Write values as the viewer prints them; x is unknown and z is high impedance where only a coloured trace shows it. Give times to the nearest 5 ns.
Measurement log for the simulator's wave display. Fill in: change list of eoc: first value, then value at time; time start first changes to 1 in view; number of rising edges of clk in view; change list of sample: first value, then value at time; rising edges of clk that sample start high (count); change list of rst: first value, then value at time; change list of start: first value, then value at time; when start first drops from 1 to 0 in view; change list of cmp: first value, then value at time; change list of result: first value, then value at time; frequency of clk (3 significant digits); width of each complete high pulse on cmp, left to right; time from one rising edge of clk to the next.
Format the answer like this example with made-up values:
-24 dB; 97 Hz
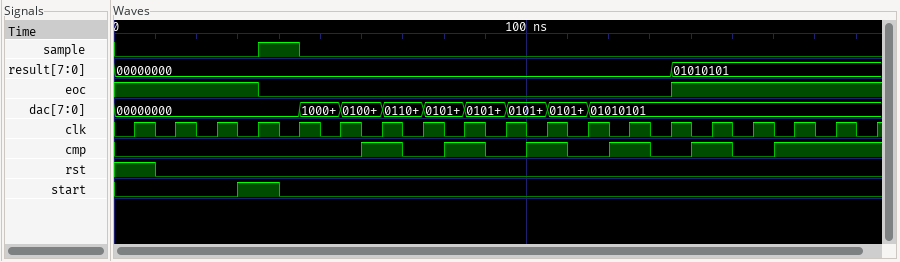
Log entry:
1, 0 at 35 ns, 1 at 135 ns; 30 ns; 19; 0, 1 at 35 ns, 0 at 45 ns; 1; 1, 0 at 10 ns; 0, 1 at 30 ns, 0 at 40 ns; 40 ns; 0, 1 at 60 ns, 0 at 70 ns, 1 at 80 ns, 0 at 90 ns, 1 at 100 ns, 0 at 110 ns, 1 at 120 ns, 0 at 130 ns, 1 at 140 ns, 0 at 150 ns, 1 at 160 ns; 00000000, 01010101 at 135 ns; 100 MHz; 10 ns, 10 ns, 10 ns, 10 ns, 10 ns; 10 ns
